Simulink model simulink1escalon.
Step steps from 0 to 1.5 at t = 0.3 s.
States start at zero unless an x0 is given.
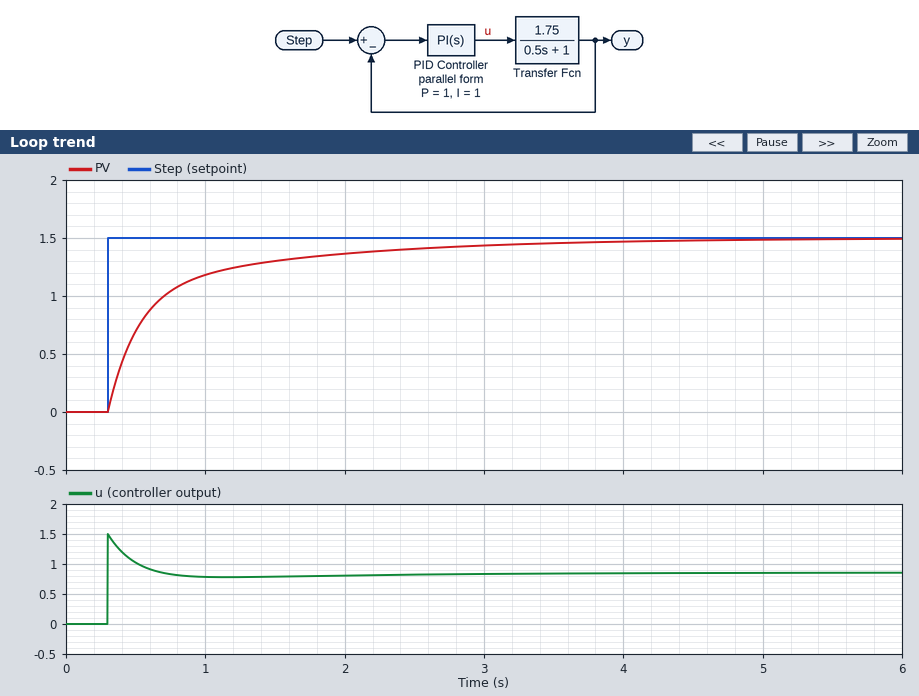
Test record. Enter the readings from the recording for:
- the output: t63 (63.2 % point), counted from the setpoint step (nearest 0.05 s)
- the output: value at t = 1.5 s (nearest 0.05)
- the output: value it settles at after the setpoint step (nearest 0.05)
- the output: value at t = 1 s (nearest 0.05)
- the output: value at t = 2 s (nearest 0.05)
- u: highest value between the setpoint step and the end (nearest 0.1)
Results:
0.35 s
1.30
1.50
1.20
1.35
1.5
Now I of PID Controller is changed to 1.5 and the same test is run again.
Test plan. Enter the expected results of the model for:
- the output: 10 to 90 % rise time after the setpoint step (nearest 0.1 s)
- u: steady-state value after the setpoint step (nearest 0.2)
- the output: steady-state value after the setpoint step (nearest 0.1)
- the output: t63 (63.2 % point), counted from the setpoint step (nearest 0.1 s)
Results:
0.9 s
0.8
1.5
0.3 s
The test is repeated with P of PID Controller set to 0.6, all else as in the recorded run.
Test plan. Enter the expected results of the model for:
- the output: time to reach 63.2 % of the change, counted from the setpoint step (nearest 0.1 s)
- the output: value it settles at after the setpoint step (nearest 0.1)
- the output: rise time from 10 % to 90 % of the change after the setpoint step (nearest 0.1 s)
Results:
0.5 s
1.5
1.3 s
